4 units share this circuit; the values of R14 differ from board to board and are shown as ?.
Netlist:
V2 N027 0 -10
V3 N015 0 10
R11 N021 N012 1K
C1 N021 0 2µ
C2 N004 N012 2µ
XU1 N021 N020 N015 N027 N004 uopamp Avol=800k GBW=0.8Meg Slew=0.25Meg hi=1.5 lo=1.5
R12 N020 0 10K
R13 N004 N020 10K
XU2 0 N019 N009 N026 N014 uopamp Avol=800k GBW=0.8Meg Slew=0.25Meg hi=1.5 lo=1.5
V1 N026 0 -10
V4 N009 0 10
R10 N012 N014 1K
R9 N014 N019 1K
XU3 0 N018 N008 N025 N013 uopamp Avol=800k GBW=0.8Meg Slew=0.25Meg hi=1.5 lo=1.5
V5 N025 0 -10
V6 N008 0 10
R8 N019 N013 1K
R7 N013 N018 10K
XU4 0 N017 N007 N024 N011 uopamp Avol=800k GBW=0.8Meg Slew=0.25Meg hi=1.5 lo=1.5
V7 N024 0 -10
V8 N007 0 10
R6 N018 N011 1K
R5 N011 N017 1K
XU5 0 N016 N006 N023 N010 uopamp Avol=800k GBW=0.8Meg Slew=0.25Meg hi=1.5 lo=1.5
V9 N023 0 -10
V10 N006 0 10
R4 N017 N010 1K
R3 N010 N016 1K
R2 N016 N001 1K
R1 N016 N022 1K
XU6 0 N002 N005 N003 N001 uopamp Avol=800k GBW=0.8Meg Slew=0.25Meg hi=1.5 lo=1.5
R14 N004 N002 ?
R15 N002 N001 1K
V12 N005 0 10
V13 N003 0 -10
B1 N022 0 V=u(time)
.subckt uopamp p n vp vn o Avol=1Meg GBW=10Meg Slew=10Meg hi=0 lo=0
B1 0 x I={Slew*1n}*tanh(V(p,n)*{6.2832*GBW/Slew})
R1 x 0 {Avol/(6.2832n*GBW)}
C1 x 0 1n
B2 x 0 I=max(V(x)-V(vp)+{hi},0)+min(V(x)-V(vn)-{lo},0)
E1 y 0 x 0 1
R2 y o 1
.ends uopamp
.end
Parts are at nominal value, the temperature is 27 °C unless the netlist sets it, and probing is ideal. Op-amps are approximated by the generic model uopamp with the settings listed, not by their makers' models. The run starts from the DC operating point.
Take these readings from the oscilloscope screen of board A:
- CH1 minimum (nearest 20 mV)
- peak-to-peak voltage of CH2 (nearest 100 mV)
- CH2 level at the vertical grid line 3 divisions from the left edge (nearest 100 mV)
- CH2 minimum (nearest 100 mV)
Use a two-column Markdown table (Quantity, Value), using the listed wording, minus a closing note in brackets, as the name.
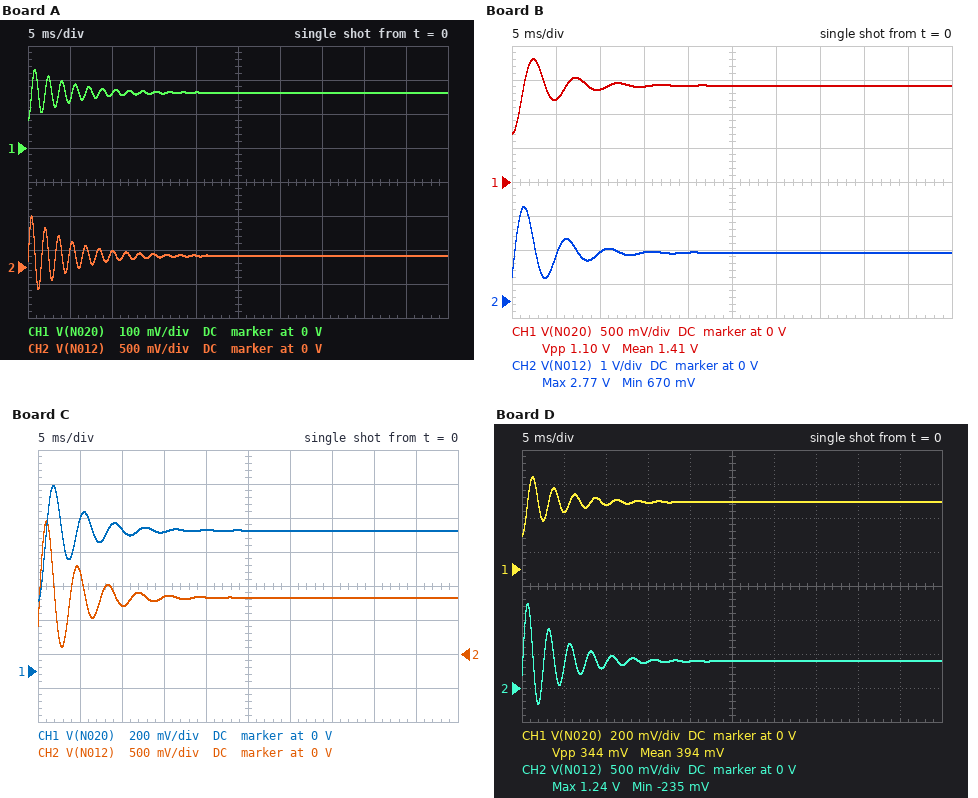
| Quantity | Value |
|---|---|
| CH1 minimum | 80 mV |
| peak-to-peak voltage of CH2 | 1.1 V |
| CH2 level at the vertical grid line 3 divisions from the left edge | 200 mV |
| CH2 minimum | -300 mV |
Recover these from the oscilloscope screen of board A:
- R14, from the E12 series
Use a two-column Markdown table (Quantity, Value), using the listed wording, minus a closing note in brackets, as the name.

| Quantity | Value |
|---|---|
| R14, from the E12 series | 330 Ω |
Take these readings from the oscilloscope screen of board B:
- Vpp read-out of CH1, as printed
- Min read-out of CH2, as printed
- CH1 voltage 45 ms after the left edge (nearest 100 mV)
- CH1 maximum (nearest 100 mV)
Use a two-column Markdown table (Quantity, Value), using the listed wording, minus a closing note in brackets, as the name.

| Quantity | Value |
|---|---|
| Vpp read-out of CH1, as printed | 1.10 V |
| Min read-out of CH2, as printed | 670 mV |
| CH1 voltage 45 ms after the left edge | 1.4 V |
| CH1 maximum | 1.8 V |
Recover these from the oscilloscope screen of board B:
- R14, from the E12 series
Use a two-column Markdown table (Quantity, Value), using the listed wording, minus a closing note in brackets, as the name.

| Quantity | Value |
|---|---|
| R14, from the E12 series | 3.3 kΩ |
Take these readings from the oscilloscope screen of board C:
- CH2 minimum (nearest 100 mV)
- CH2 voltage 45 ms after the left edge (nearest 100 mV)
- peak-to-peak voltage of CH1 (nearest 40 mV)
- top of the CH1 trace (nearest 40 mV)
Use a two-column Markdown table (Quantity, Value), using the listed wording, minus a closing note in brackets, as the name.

| Quantity | Value |
|---|---|
| CH2 minimum | 100 mV |
| CH2 voltage 45 ms after the left edge | 800 mV |
| peak-to-peak voltage of CH1 | 680 mV |
| top of the CH1 trace | 1.08 V |
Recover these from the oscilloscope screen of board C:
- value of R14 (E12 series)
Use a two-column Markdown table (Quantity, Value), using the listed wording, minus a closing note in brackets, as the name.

| Quantity | Value |
|---|---|
| value of R14 | 1.8 kΩ |
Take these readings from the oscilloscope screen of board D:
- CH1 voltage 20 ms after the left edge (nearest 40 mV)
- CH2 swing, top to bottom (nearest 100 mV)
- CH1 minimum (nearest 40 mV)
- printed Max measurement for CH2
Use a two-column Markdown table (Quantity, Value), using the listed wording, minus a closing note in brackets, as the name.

| Quantity | Value |
|---|---|
| CH1 voltage 20 ms after the left edge | 400 mV |
| CH2 swing, top to bottom | 1.5 V |
| CH1 minimum | 200 mV |
| printed Max measurement for CH2 | 1.24 V |
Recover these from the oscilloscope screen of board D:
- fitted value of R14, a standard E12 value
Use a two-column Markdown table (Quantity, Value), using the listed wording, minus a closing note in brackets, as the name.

| Quantity | Value |
|---|---|
| fitted value of R14, a standard E12 value | 820 Ω |
